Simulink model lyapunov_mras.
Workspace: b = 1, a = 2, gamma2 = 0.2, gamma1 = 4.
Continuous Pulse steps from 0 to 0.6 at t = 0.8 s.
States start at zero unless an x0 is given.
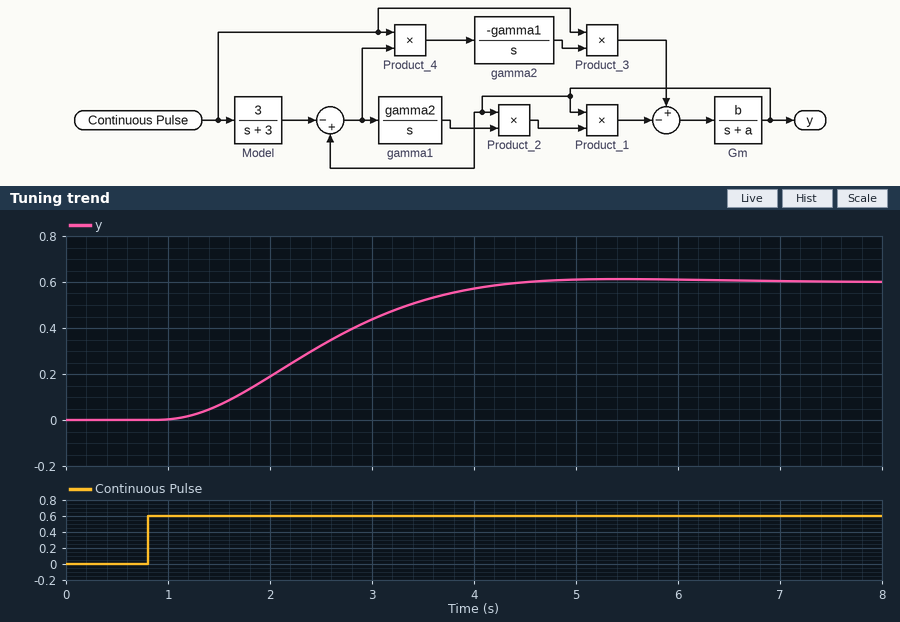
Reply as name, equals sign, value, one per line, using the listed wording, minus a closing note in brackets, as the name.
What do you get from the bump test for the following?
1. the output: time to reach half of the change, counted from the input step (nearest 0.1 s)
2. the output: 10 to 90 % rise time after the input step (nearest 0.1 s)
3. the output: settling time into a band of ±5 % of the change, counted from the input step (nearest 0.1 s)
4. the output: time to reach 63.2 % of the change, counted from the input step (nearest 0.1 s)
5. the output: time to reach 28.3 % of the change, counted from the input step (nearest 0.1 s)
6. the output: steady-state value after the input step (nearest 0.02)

the output: time to reach half of the change, counted from the input step = 1.6 s
the output: 10 to 90 % rise time after the input step = 2.2 s
the output: settling time into a band of ±5 % of the change, counted from the input step = 3.2 s
the output: time to reach 63.2 % of the change, counted from the input step = 1.9 s
the output: time to reach 28.3 % of the change, counted from the input step = 1.1 s
the output: steady-state value after the input step = 0.60
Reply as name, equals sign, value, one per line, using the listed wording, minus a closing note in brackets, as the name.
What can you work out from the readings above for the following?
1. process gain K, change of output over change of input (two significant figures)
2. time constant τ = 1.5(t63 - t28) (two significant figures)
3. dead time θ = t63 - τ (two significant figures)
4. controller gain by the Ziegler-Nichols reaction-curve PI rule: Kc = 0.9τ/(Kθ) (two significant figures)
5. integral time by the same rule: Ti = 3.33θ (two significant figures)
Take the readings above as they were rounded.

process gain K, change of output over change of input = 1.0
time constant τ = 1.5(t63 - t28) = 1.2 s
dead time θ = t63 - τ = 0.70 s
controller gain by the Ziegler-Nichols reaction-curve PI rule: Kc = 0.9τ/(Kθ) = 1.5
integral time by the same rule: Ti = 3.33θ = 2.3 s
